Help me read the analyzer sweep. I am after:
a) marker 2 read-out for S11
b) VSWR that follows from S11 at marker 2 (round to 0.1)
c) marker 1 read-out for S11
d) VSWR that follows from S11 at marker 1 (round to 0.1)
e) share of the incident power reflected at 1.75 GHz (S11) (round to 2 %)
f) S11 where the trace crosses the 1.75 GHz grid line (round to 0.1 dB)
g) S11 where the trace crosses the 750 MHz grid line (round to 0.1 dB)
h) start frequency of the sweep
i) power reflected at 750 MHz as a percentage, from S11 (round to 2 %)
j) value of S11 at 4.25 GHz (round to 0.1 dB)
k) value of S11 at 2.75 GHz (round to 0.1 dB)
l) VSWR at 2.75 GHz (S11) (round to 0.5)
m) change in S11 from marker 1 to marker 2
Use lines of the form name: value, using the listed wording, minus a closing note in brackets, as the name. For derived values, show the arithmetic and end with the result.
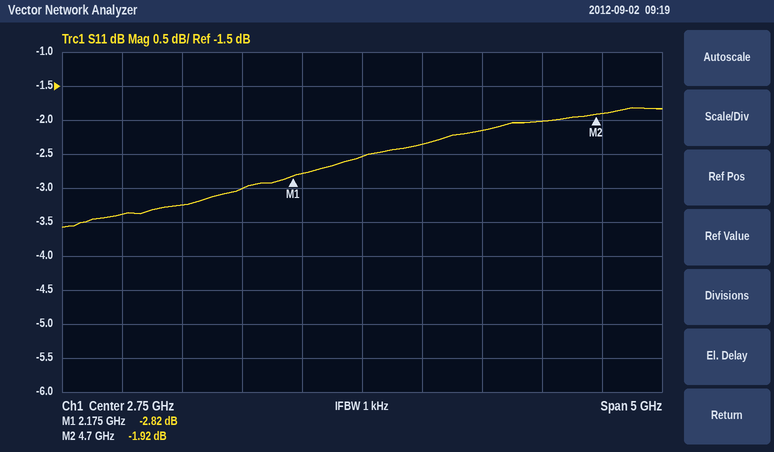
marker 2 read-out for S11: -1.92 dB
VSWR that follows from S11 at marker 2: (1 + 0.8017)/(1 − 0.8017) ≈ 9.1
marker 1 read-out for S11: -2.82 dB
VSWR that follows from S11 at marker 1: (1 + 0.7228)/(1 − 0.7228) ≈ 6.2
share of the incident power reflected at 1.75 GHz (S11): 10^(-3/10) ≈ 50 %
S11 where the trace crosses the 1.75 GHz grid line: -3.0 dB
S11 where the trace crosses the 750 MHz grid line: -3.4 dB
start frequency of the sweep: 250 MHz
power reflected at 750 MHz as a percentage, from S11: 10^(-3.4/10) ≈ 46 %
value of S11 at 4.25 GHz: -2.0 dB
value of S11 at 2.75 GHz: -2.5 dB
VSWR at 2.75 GHz (S11): |Γ| = 10^(-2.5/20) = 0.7499; VSWR = (1 + 0.7499)/(1 − 0.7499) ≈ 7.0
change in S11 from marker 1 to marker 2: -1.92 − (-2.82) = 0.90 dB
